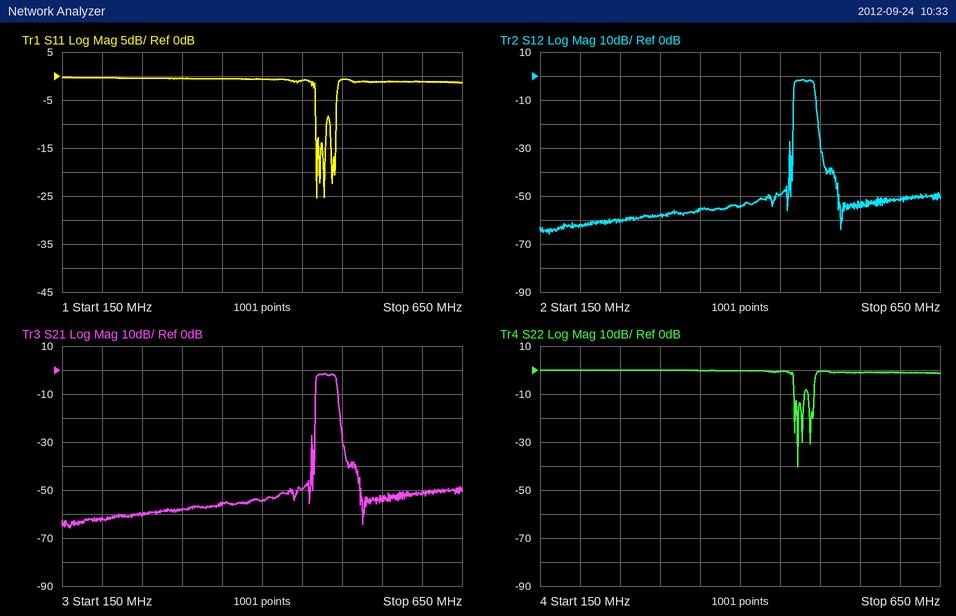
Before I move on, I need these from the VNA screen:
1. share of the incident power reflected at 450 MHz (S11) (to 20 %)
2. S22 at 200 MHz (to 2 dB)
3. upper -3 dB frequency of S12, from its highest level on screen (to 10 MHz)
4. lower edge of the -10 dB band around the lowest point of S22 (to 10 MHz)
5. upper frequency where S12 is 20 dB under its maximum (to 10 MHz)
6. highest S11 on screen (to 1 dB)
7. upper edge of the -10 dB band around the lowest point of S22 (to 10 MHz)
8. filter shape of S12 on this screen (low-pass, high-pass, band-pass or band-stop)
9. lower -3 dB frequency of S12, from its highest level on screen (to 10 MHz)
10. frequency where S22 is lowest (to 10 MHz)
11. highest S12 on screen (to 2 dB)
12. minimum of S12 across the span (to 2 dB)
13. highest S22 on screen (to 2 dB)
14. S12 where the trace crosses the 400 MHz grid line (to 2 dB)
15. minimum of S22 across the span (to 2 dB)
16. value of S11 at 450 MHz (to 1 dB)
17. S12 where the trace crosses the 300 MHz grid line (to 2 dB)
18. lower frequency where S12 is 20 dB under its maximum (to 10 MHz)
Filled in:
80 %
0 dB
490 MHz
470 MHz
500 MHz
0 dB
480 MHz
band-pass
470 MHz
470 MHz
-2 dB
-66 dB
0 dB
-54 dB
-40 dB
-1 dB
-58 dB
470 MHz
